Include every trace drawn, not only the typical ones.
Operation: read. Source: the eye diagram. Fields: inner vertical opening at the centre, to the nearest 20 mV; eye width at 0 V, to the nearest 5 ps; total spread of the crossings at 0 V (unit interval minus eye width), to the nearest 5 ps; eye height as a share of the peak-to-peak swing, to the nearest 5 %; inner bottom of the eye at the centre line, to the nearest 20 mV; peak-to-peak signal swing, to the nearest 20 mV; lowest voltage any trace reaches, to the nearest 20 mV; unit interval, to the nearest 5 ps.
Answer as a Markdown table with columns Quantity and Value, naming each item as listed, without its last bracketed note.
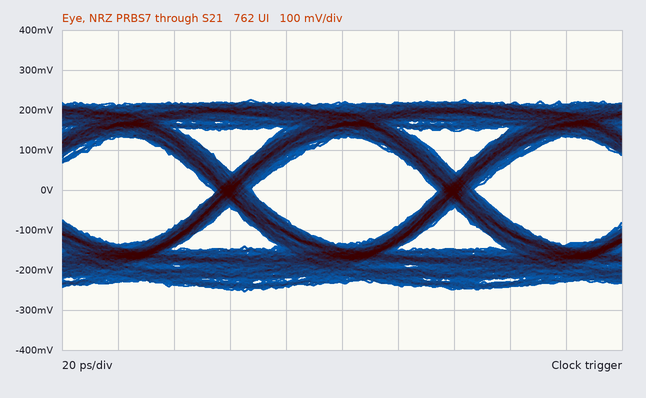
| Quantity | Value |
|---|---|
| inner vertical opening at the centre, to the nearest 20 mV | 260 mV |
| eye width at 0 V, to the nearest 5 ps | 65 ps |
| total spread of the crossings at 0 V (unit interval minus eye width), to the nearest 5 ps | 15 ps |
| eye height as a share of the peak-to-peak swing, to the nearest 5 % | 55 % |
| inner bottom of the eye at the centre line, to the nearest 20 mV | -140 mV |
| peak-to-peak signal swing, to the nearest 20 mV | 480 mV |
| lowest voltage any trace reaches, to the nearest 20 mV | -260 mV |
| unit interval, to the nearest 5 ps | 80 ps |
